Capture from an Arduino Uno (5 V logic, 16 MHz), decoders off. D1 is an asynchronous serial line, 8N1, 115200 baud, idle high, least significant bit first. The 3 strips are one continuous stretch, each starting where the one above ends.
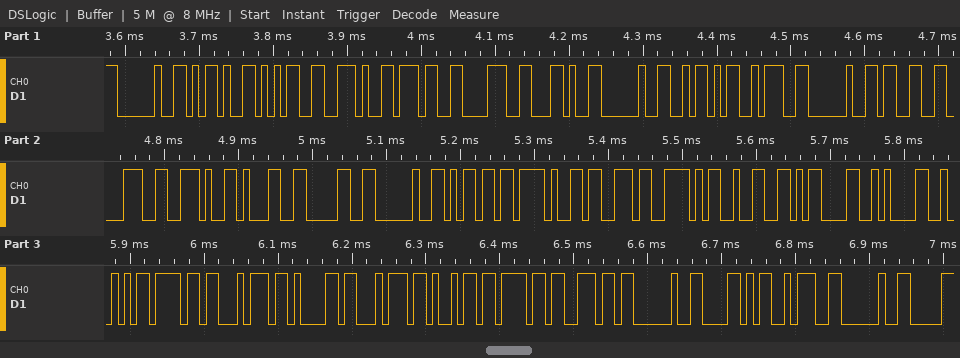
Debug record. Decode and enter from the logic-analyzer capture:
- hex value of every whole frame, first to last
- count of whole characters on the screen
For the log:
20 2D 35 2E 37 38 2C 20 5A 3A 20 33 38 2E 31 30 20 6D 2F 73 5E 32 0D 0A 52 6F 74 61 74 69 6F 6E 20 58 3A 20
36
